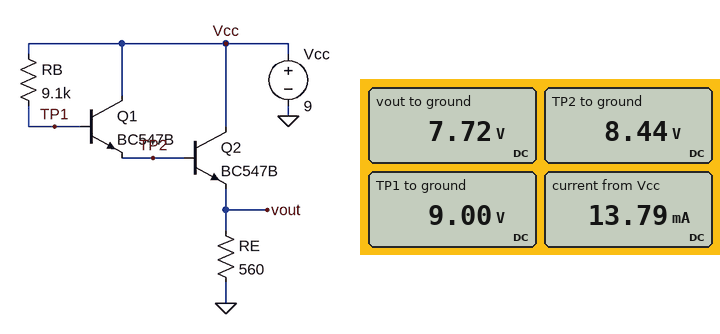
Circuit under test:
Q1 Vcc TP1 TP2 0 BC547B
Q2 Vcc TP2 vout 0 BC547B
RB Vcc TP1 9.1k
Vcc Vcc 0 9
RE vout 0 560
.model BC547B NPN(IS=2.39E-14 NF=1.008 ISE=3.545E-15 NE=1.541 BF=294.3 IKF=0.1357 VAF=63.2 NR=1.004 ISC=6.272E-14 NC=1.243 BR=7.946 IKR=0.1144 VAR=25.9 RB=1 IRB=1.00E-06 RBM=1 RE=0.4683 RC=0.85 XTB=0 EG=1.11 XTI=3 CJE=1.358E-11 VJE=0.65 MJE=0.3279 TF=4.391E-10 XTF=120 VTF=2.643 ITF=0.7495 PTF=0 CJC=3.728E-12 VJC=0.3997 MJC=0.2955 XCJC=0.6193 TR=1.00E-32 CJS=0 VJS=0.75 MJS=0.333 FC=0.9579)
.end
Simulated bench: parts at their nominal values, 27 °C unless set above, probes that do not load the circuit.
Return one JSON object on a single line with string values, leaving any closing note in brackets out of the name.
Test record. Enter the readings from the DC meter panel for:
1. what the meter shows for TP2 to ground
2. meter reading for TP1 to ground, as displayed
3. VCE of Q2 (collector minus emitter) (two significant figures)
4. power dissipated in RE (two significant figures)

{"what the meter shows for TP2 to ground": "8.44 V", "meter reading for TP1 to ground, as displayed": "9.00 V", "VCE of Q2 (collector minus emitter)": "1.3 V", "power dissipated in RE": "110 mW"}
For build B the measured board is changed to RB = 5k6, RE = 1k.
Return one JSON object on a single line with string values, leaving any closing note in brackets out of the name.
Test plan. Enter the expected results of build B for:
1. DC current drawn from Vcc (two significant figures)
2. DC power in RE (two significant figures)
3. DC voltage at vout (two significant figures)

{"DC current drawn from Vcc": "7.8 mA", "DC power in RE": "60 mW", "DC voltage at vout": "7.8 V"}
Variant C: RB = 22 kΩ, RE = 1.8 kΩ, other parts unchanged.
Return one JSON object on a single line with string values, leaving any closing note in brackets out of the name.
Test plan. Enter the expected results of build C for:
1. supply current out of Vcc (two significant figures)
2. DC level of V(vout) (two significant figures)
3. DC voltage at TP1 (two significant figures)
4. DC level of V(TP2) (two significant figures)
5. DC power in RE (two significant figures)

{"supply current out of Vcc": "4.3 mA", "DC level of V(vout)": "7.8 V", "DC voltage at TP1": "9.0 V", "DC level of V(TP2)": "8.5 V", "DC power in RE": "34 mW"}
